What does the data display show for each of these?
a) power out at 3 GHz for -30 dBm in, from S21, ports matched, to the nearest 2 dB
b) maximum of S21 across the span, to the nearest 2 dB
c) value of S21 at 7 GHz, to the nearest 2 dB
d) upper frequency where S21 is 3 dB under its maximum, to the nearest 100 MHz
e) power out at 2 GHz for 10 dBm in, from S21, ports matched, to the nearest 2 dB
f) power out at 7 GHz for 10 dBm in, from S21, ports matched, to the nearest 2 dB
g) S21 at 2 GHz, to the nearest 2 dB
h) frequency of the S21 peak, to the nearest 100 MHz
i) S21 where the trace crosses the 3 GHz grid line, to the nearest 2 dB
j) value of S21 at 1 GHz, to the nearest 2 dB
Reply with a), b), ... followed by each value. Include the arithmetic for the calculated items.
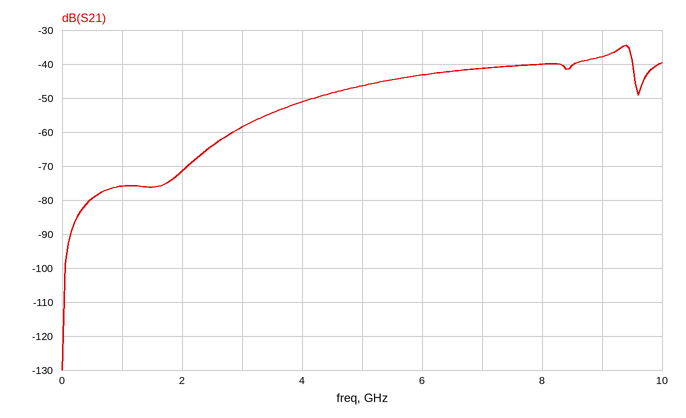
a) -30 dBm + (-58 dB) = -88 dBm
b) -34 dB
c) -42 dB
d) 9.5 GHz
e) 10 dBm + (-72 dB) = -62 dBm
f) 10 dBm + (-42 dB) = -32 dBm
g) -72 dB
h) 9.4 GHz
i) -58 dB
j) -76 dB
